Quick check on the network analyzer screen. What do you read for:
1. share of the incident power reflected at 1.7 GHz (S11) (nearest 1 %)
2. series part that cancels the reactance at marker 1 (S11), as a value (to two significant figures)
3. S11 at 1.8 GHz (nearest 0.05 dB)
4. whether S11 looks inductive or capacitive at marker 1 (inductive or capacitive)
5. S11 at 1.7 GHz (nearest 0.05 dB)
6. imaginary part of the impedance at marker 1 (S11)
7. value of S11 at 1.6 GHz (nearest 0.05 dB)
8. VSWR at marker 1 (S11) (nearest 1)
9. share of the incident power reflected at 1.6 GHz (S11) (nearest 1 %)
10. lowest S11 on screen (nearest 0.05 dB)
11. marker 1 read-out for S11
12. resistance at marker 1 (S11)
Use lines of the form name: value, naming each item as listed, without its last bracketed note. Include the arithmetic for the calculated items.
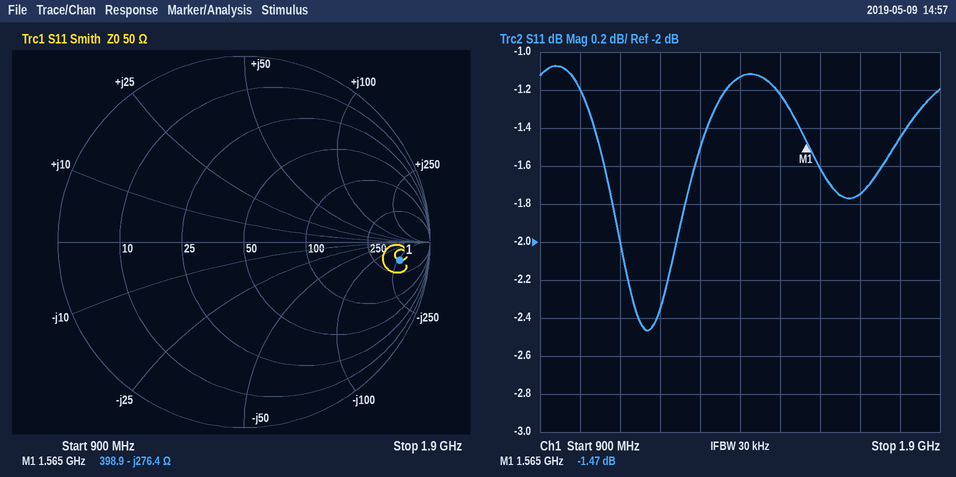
share of the incident power reflected at 1.7 GHz (S11): 10^(-1.75/10) ≈ 67 %
series part that cancels the reactance at marker 1 (S11), as a value: L = 276.4 Ω/(2π × 1.565 GHz) ≈ 28 nH
S11 at 1.8 GHz: -1.45 dB
whether S11 looks inductive or capacitive at marker 1: capacitive
S11 at 1.7 GHz: -1.75 dB
imaginary part of the impedance at marker 1: -276.4 Ω
value of S11 at 1.6 GHz: -1.60 dB
VSWR at marker 1 (S11): (1 + 0.8443)/(1 − 0.8443) ≈ 12
share of the incident power reflected at 1.6 GHz (S11): 10^(-1.6/10) ≈ 69 %
lowest S11 on screen: -2.45 dB
marker 1 read-out for S11: -1.47 dB
resistance at marker 1: 398.9 Ω
